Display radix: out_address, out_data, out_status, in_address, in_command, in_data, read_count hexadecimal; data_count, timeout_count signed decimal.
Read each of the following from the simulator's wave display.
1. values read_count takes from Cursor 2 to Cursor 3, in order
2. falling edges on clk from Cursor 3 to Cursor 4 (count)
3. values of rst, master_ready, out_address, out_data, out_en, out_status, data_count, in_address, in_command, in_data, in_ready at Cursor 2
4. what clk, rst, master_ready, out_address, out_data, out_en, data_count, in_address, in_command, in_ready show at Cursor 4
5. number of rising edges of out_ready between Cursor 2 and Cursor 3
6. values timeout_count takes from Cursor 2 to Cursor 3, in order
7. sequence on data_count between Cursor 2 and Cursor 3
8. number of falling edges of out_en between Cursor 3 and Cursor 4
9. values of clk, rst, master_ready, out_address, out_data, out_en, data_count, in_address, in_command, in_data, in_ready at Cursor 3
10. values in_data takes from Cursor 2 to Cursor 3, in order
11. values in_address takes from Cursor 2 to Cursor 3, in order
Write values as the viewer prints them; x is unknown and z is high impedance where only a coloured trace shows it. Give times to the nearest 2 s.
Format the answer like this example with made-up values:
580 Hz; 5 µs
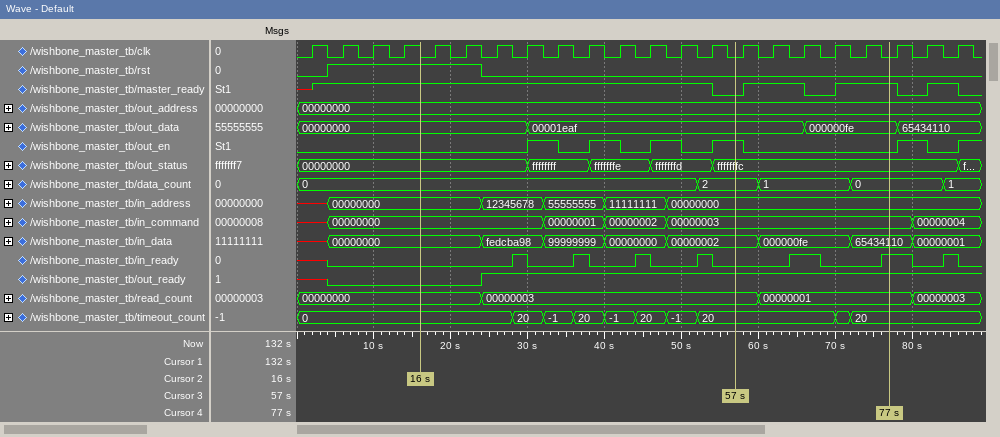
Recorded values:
00000000, 00000003; 5; rst=1, master_ready=1, out_address=00000000, out_data=00000000, out_en=0, out_status=00000000, data_count=0, in_address=00000000, in_command=00000000, in_data=00000000, in_ready=0; clk=0, rst=0, master_ready=1, out_address=00000000, out_data=000000fe, out_en=0, data_count=0, in_address=00000000, in_command=00000003, in_ready=1; 1; 0, 20, -1, 20, -1, 20, -1, 20; 0, 2; 1; clk=0, rst=0, master_ready=0, out_address=00000000, out_data=00001eaf, out_en=1, data_count=2, in_address=00000000, in_command=00000003, in_data=00000002, in_ready=0; 00000000, fedcba98, 99999999, 00000000, 00000002; 00000000, 12345678, 55555555, 11111111, 00000000
